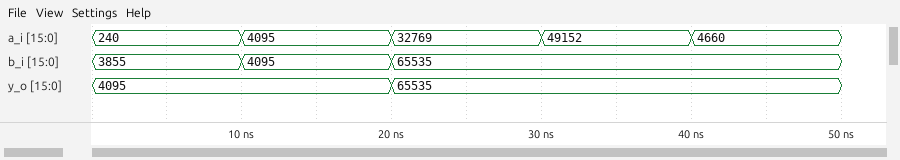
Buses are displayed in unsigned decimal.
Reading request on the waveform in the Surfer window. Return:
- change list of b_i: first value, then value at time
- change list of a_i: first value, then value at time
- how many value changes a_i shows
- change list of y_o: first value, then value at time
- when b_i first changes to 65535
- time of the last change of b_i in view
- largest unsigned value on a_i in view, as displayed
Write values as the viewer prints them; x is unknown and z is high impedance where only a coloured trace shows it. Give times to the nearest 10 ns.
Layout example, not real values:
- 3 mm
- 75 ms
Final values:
- 3855, 4095 at 10 ns, 65535 at 20 ns
- 240, 4095 at 10 ns, 32769 at 20 ns, 49152 at 30 ns, 4660 at 40 ns
- 4
- 4095, 65535 at 20 ns
- 20 ns
- 20 ns
- 49152
